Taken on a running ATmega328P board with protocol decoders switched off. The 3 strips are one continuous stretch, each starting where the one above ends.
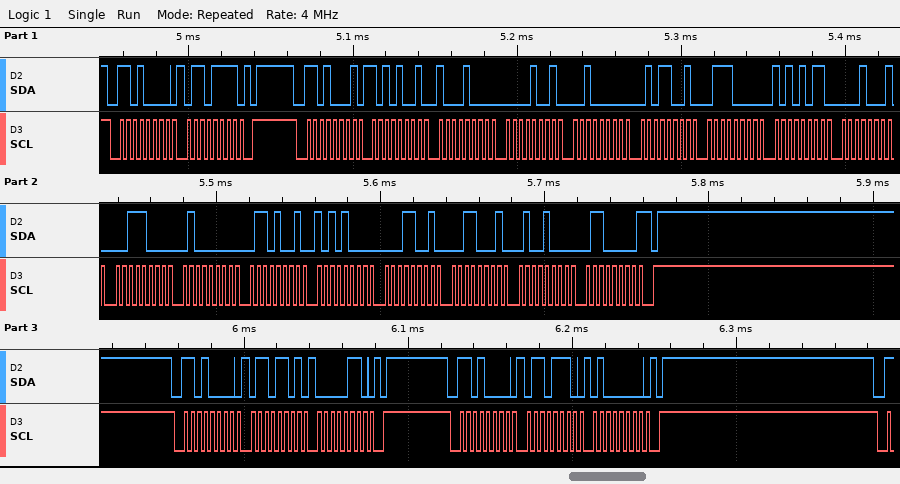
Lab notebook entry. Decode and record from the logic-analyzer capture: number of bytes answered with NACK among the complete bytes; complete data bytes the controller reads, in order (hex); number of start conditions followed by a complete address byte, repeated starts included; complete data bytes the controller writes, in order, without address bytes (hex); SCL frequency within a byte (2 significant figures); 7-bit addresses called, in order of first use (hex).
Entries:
1
A9 88 09 20 59 70 AB 11 38 40 69 A8 19 31 48 60
4
6F 6D 06 6E 40
250 kHz
0x68
